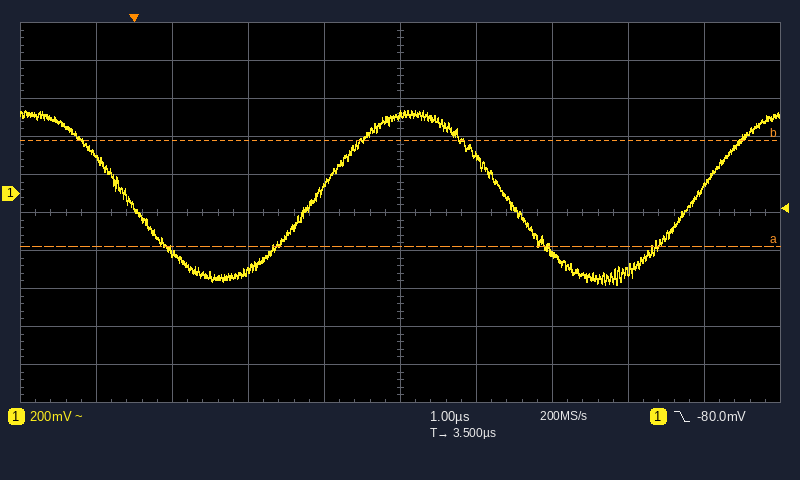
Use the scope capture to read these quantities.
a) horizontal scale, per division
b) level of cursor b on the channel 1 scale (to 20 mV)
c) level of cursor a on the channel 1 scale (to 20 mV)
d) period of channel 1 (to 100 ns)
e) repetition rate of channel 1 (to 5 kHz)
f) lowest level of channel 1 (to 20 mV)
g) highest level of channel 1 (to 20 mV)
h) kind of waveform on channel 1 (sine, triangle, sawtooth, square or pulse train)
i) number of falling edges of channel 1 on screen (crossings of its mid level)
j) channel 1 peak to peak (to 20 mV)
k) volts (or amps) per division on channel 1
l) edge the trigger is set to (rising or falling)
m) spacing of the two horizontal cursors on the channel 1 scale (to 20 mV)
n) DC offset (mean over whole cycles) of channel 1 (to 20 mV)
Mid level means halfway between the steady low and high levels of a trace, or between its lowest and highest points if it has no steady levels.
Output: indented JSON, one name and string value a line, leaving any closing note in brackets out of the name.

{
  "horizontal scale, per division": "1 µs",
  "level of cursor b on the channel 1 scale": "280 mV",
  "level of cursor a on the channel 1 scale": "-280 mV",
  "period of channel 1": "5.0 µs",
  "repetition rate of channel 1": "200 kHz",
  "lowest level of channel 1": "-480 mV",
  "highest level of channel 1": "440 mV",
  "kind of waveform on channel 1": "sine",
  "number of falling edges of channel 1 on screen": "2",
  "channel 1 peak to peak": "920 mV",
  "volts (or amps) per division on channel 1": "200 mV",
  "edge the trigger is set to": "falling",
  "spacing of the two horizontal cursors on the channel 1 scale": "560 mV",
  "DC offset (mean over whole cycles) of channel 1": "-20 mV"
}
